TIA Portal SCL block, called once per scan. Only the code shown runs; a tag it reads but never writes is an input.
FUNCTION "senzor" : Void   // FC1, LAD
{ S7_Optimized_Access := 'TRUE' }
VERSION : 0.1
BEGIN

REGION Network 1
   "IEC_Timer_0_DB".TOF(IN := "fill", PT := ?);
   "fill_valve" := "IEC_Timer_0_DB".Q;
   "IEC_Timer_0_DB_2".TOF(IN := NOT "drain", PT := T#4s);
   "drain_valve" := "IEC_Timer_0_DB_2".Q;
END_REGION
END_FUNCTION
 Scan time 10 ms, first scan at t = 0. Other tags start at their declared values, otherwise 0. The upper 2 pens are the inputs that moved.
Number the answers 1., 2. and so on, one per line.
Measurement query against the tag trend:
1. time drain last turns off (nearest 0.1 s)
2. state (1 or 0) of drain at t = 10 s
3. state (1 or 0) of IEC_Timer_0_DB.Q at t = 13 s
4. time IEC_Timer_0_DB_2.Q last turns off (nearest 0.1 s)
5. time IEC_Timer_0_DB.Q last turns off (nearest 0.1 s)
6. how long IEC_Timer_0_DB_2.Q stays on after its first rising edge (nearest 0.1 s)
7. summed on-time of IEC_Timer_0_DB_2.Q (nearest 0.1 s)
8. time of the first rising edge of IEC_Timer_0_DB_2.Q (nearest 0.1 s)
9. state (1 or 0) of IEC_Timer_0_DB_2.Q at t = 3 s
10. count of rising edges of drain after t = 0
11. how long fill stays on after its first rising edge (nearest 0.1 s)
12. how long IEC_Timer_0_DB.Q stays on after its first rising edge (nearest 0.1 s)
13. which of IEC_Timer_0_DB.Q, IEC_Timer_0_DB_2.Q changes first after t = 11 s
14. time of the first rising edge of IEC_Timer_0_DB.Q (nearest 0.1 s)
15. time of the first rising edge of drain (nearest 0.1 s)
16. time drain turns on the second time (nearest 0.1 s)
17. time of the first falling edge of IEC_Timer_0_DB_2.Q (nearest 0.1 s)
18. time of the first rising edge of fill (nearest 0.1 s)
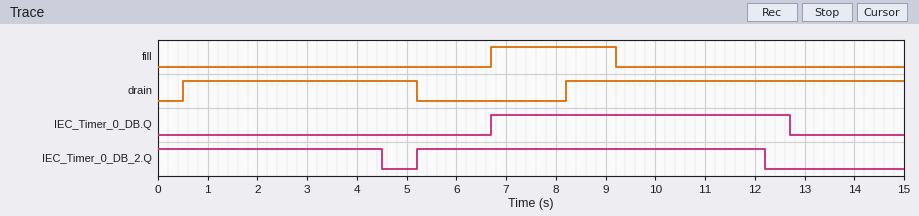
1. 5.2 s
2. 1
3. 0
4. 12.2 s
5. 12.7 s
6. 7.0 s
7. 11.5 s
8. 5.2 s
9. 1
10. 2
11. 2.5 s
12. 6.0 s
13. IEC_Timer_0_DB_2.Q
14. 6.7 s
15. 0.5 s
16. 8.2 s
17. 4.5 s
18. 6.7 s
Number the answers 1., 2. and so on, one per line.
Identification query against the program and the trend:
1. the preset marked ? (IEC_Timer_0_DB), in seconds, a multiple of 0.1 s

1. 3.5 s
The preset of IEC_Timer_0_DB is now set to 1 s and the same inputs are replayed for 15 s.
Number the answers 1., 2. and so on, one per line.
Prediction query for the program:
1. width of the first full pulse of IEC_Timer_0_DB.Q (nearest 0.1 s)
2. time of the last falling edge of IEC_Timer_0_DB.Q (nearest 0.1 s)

1. 3.5 s
2. 10.2 s
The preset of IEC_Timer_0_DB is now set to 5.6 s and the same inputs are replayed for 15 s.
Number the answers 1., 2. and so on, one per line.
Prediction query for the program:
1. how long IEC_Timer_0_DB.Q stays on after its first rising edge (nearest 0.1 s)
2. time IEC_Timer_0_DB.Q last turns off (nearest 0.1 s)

1. 8.1 s
2. 14.8 s
